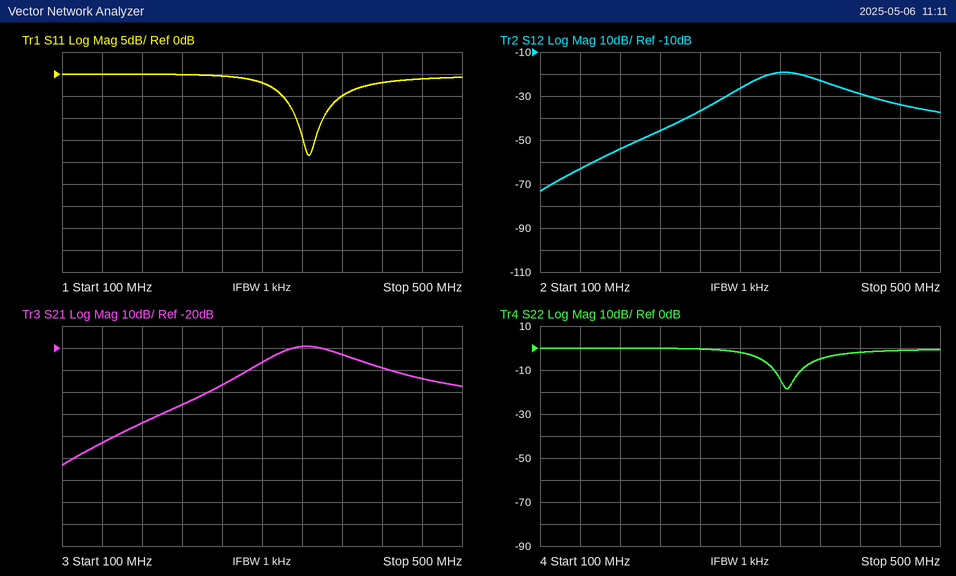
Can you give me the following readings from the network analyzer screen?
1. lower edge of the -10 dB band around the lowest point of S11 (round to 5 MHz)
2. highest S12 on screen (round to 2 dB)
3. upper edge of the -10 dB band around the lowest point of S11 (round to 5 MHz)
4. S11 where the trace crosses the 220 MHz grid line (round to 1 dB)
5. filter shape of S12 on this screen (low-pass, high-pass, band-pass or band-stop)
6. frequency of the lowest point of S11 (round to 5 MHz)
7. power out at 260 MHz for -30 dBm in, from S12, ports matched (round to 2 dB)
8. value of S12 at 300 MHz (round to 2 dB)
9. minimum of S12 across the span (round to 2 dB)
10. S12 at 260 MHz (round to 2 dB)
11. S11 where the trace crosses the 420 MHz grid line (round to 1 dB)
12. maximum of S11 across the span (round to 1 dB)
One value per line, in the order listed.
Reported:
335 MHz
-20 dB
360 MHz
0 dB
band-pass
345 MHz
-66 dBm
-26 dB
-74 dB
-36 dB
-2 dB
0 dB
